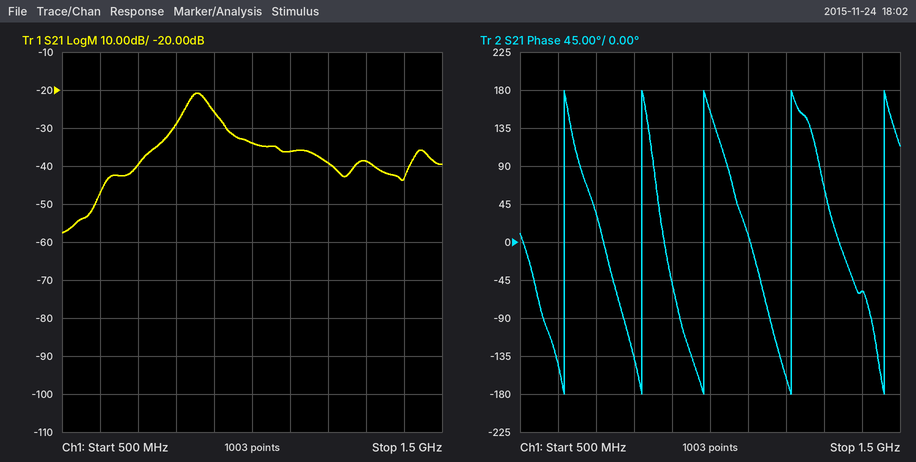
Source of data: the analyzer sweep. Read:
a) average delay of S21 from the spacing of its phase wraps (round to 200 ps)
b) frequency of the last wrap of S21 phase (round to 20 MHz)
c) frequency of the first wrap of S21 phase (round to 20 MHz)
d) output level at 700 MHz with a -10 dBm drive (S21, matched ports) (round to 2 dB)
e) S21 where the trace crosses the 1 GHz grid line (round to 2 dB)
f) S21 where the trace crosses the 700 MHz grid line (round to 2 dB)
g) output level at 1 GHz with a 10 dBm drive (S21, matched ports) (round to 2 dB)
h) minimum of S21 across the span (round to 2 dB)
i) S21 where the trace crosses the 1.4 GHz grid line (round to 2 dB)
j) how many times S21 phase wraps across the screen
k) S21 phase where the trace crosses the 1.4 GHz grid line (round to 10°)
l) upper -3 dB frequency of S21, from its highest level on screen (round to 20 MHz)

4.8 ns
1.46 GHz
620 MHz
-50 dBm
-34 dB
-40 dB
-24 dBm
-58 dB
-44 dB
5
-60°
880 MHz
